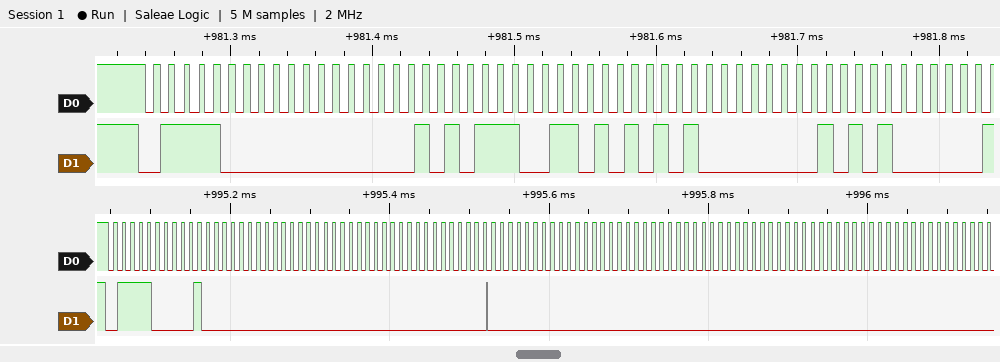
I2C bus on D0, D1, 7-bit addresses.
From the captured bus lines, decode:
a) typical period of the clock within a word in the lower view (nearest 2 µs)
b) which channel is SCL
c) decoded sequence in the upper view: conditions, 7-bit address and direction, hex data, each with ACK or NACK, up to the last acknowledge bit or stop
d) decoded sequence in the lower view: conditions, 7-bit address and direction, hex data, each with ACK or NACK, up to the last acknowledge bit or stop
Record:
10 µs
D0
start, address 3C write ACK, 00 ACK, AE ACK, D5 ACK, 80 ACK, A8 ACK
start, address 3C write ACK, 40 ACK, 00 ACK, 00 ACK, 00 ACK, 00 ACK, 00 ACK, 00 ACK, 00 ACK, 00 ACK, 00 ACK
